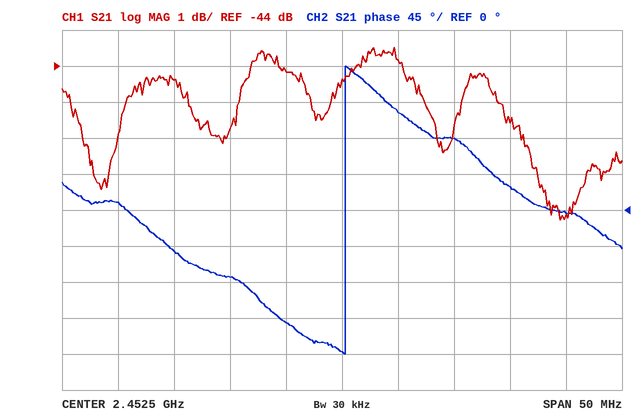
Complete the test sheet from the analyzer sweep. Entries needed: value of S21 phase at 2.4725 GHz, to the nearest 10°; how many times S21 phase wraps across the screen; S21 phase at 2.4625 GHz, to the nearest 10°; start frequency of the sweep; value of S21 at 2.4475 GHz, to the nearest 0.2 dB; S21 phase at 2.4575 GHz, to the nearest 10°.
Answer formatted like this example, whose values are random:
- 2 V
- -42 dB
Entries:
- 0°
- 1
- 90°
- 2.4275 GHz
- -44.2 dB
- 120°
